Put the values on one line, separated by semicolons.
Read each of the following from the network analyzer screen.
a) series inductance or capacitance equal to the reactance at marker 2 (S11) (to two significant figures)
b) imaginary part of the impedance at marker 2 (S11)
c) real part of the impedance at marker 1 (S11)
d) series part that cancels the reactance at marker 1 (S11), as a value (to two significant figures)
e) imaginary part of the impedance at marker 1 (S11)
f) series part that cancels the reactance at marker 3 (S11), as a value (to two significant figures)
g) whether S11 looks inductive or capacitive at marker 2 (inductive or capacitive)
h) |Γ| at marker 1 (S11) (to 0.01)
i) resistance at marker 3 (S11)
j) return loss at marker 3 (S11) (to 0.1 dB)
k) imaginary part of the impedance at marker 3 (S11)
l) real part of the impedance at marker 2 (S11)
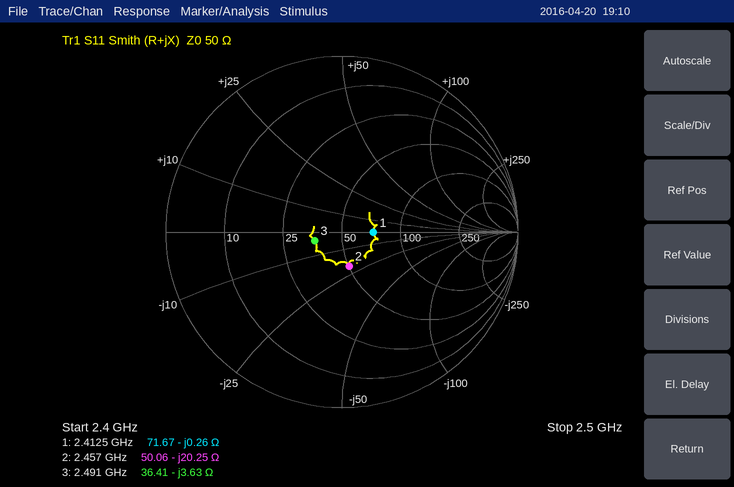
3.2 pF; -20.25 Ω; 71.67 Ω; 17 pH; -0.26 Ω; 230 pH; capacitive; 0.18; 36.41 Ω; 15.8 dB; -3.63 Ω; 50.06 Ω
